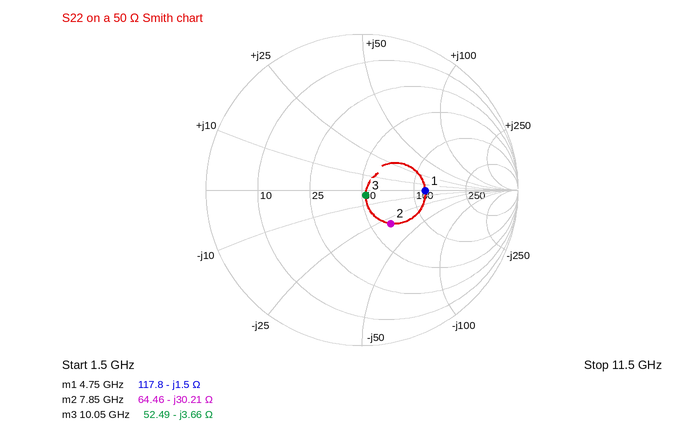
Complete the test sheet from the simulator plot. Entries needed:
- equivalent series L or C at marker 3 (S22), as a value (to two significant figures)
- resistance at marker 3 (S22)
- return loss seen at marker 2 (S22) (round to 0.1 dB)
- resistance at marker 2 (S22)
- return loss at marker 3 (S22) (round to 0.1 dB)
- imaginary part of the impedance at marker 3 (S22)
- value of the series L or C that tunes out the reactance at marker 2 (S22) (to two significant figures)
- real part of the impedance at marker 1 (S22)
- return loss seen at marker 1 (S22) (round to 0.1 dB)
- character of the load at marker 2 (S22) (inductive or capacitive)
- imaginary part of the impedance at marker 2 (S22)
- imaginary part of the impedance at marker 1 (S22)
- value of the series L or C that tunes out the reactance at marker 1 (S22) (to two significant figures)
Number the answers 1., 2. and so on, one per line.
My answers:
1. 4.3 pF
2. 52.49 Ω
3. 11.0 dB
4. 64.46 Ω
5. 27.3 dB
6. -3.66 Ω
7. 610 pH
8. 117.8 Ω
9. 7.9 dB
10. capacitive
11. -30.21 Ω
12. -1.5 Ω
13. 50 pH
